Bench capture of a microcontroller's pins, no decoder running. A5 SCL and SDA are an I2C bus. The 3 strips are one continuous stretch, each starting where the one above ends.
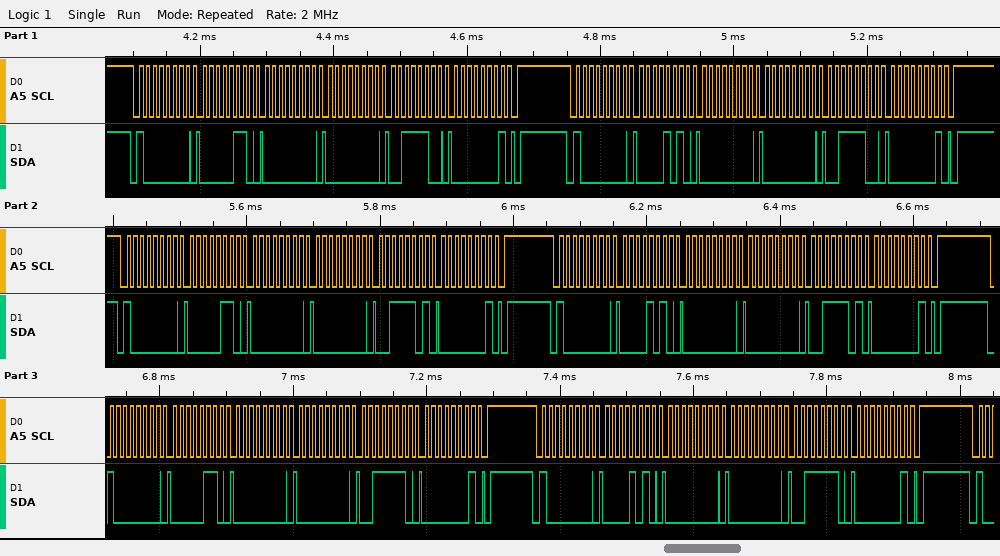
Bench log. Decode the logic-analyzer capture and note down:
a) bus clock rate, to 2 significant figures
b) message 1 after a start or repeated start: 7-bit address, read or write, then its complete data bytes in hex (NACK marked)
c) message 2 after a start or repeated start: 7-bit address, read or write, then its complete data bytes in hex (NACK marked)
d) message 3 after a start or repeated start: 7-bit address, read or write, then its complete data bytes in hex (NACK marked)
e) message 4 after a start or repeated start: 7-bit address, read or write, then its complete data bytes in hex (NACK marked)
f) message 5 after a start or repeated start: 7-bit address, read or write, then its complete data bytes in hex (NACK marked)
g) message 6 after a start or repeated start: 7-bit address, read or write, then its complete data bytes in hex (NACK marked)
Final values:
100 kHz
0x40 write: 06 00 00 3C 01
0x40 write: 0A 00 00 3C 01
0x40 write: 06 00 00 3D 01
0x40 write: 0A 00 00 3D 01
0x40 write: 06 00 00 3E 01
0x40 write: 0A 00 00 3E 01
